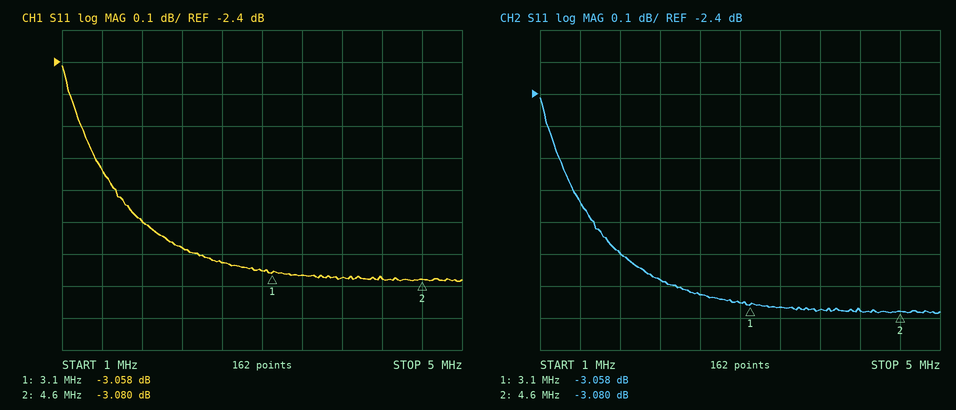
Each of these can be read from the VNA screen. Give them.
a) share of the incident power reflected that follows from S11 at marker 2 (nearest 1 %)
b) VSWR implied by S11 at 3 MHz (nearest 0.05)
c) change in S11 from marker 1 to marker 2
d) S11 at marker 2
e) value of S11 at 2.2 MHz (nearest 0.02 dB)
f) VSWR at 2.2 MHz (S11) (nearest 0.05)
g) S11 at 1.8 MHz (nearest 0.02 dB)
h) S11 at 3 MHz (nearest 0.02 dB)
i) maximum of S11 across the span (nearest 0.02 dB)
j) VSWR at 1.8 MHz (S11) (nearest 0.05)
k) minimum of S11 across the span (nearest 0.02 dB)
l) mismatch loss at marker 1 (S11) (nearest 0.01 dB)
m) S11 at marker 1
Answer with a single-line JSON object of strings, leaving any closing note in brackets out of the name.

{"share of the incident power reflected that follows from S11 at marker 2": "49 %", "VSWR implied by S11 at 3 MHz": "5.75", "change in S11 from marker 1 to marker 2": "-0.022 dB", "S11 at marker 2": "-3.080 dB", "value of S11 at 2.2 MHz": "-2.98 dB", "VSWR at 2.2 MHz (S11)": "5.90", "S11 at 1.8 MHz": "-2.90 dB", "S11 at 3 MHz": "-3.06 dB", "maximum of S11 across the span": "-2.42 dB", "VSWR at 1.8 MHz (S11)": "6.05", "minimum of S11 across the span": "-3.08 dB", "mismatch loss at marker 1 (S11)": "2.96 dB", "S11 at marker 1": "-3.058 dB"}
